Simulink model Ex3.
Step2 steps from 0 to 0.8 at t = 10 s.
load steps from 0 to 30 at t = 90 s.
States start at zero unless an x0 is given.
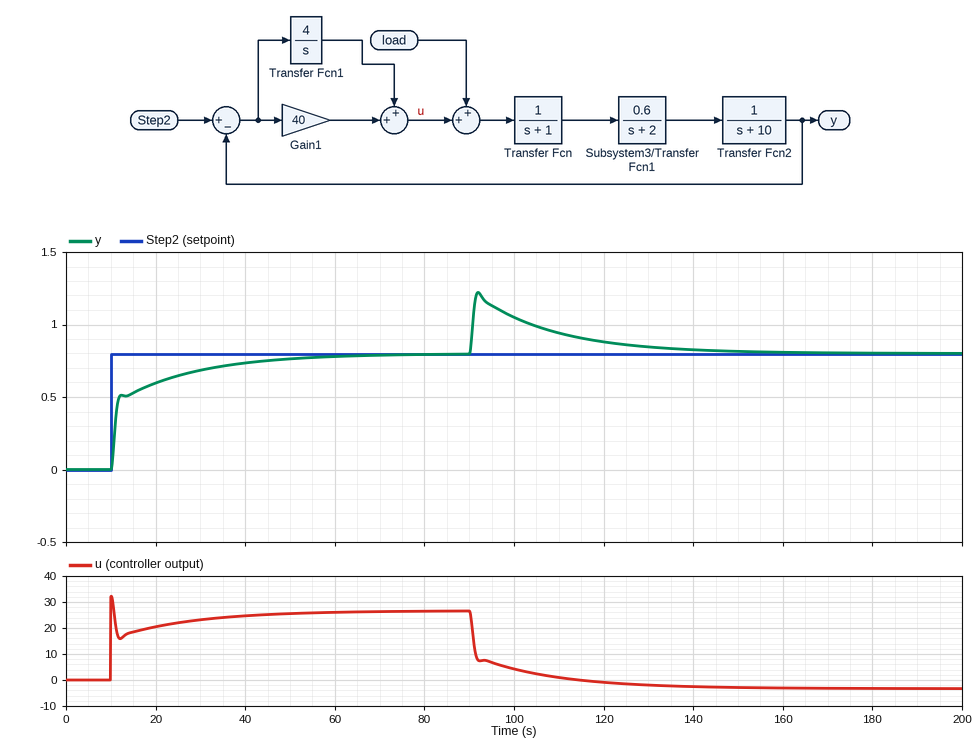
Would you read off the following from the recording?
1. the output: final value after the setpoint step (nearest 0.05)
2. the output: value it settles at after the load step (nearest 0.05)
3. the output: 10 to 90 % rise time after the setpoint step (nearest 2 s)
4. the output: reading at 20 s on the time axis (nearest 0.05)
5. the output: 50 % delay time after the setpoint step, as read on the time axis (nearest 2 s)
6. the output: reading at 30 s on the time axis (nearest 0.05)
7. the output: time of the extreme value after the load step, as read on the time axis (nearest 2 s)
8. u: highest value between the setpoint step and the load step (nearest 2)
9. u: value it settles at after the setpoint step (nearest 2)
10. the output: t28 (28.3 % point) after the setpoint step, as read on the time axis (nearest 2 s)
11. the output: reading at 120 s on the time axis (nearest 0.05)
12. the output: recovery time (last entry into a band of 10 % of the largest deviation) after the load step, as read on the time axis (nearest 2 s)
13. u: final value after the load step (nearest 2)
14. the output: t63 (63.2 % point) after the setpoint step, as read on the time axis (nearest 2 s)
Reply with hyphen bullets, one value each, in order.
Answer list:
- 0.80
- 0.80
- 26 s
- 0.60
- 12 s
- 0.70
- 92 s
- 32
- 26
- 10 s
- 0.90
- 132 s
- -4
- 12 s
